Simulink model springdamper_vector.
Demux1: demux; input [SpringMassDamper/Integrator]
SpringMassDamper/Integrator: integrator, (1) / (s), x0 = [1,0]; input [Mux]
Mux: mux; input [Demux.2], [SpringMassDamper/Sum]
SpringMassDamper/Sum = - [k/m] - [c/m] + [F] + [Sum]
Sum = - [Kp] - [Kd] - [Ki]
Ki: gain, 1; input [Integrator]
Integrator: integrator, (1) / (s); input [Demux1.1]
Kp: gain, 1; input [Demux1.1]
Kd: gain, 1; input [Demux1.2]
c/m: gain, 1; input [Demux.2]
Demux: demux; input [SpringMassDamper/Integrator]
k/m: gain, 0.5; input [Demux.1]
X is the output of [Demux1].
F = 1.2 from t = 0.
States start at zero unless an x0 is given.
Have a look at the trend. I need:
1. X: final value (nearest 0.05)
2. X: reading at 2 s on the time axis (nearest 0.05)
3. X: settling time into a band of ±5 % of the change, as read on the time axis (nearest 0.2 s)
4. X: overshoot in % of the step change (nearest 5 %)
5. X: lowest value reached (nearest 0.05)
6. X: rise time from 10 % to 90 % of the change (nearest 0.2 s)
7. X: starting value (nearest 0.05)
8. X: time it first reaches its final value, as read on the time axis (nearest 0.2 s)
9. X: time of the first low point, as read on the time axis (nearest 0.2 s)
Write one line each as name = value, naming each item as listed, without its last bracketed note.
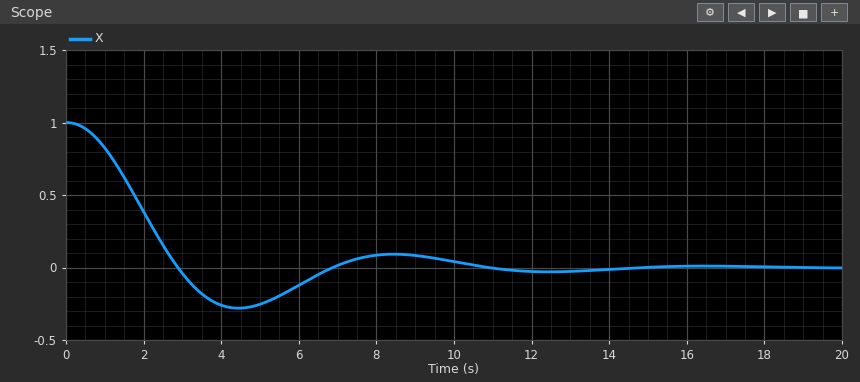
X: final value = 0.00
X: reading at 2 s on the time axis = 0.40
X: settling time into a band of ±5 % of the change, as read on the time axis = 9.8 s
X: overshoot in % of the step change = 30 %
X: lowest value reached = -0.30
X: rise time from 10 % to 90 % of the change = 1.8 s
X: starting value = 1.00
X: time it first reaches its final value, as read on the time axis = 2.8 s
X: time of the first low point, as read on the time axis = 4.4 s
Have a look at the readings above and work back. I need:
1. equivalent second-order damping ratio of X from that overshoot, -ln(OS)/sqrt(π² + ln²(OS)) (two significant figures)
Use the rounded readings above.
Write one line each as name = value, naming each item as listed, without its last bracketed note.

equivalent second-order damping ratio of X from that overshoot, -ln(OS)/sqrt(π² + ln²(OS)) = 0.36
